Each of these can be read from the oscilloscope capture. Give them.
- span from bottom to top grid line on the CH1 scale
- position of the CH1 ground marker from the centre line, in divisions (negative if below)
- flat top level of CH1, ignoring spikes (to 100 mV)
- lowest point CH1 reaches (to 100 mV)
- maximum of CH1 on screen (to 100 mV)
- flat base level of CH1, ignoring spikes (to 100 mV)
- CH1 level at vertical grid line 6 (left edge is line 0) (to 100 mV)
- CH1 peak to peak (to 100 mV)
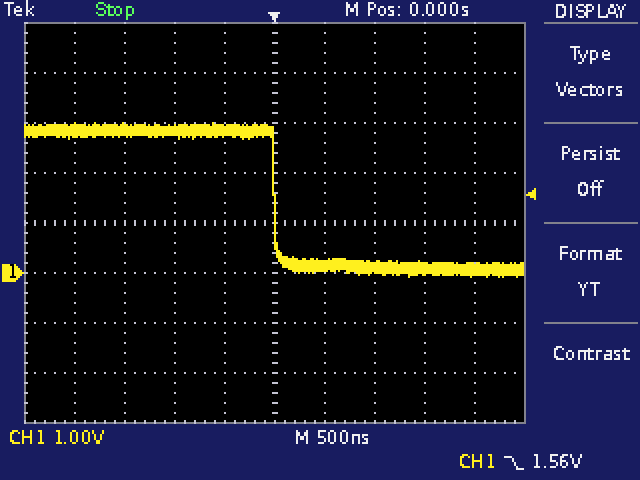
8 V
-1.0 div
2.8 V
-100 mV
3.0 V
100 mV
100 mV
3.1 V
